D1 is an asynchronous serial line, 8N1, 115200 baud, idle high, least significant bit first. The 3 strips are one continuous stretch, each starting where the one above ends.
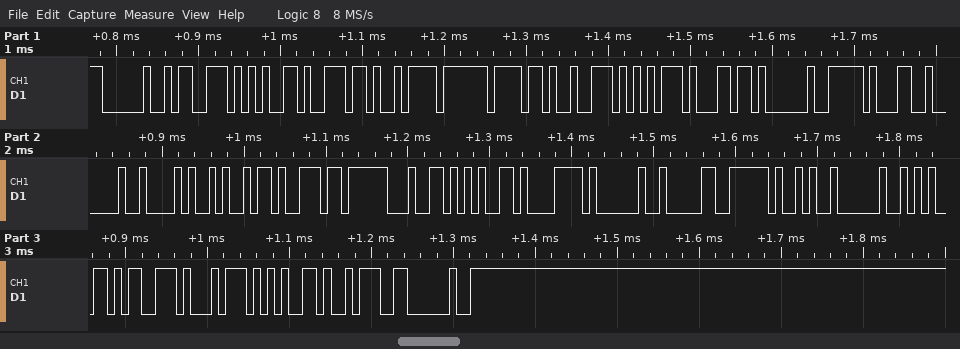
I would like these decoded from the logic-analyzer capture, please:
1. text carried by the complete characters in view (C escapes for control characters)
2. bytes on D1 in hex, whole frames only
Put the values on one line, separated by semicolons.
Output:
" senzorul 1 (index 0) este: "; 20 73 65 6E 7A 6F 72 75 6C 20 31 20 28 69 6E 64 65 78 20 30 29 20 65 73 74 65 3A 20
